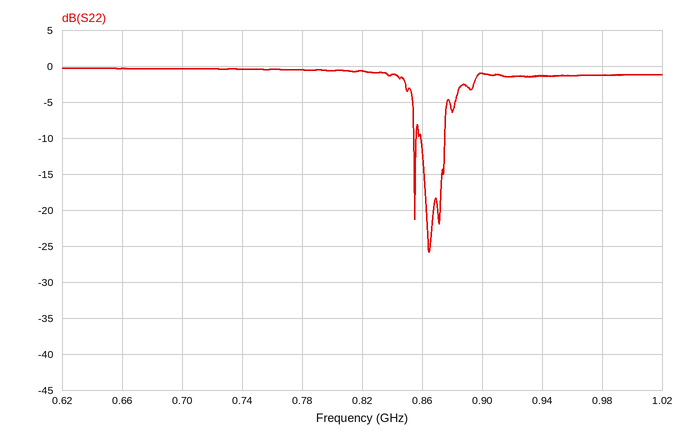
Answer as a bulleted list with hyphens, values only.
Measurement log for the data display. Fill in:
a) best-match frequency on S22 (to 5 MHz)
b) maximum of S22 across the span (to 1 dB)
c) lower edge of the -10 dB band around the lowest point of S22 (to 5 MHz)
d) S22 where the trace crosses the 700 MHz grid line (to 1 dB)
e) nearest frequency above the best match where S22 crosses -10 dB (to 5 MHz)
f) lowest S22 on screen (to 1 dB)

- 865 MHz
- 0 dB
- 860 MHz
- 0 dB
- 875 MHz
- -26 dB
